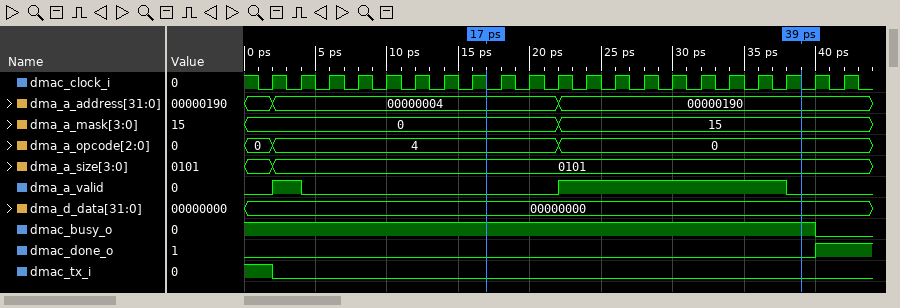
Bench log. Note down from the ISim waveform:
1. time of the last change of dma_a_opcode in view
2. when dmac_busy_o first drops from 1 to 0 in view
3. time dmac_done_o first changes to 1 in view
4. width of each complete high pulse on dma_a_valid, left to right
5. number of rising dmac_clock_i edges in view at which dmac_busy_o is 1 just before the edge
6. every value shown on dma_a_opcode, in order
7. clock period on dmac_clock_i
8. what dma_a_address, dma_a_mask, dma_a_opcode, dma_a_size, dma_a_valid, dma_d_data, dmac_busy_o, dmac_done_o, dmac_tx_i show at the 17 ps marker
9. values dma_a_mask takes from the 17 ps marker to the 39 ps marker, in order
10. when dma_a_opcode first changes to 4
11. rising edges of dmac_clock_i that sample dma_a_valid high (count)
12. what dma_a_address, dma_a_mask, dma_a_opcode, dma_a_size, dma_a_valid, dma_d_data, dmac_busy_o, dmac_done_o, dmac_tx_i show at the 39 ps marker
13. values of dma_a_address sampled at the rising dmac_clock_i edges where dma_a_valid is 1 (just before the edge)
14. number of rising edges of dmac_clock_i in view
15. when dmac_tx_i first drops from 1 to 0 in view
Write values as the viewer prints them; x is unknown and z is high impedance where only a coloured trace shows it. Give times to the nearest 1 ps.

22 ps
40 ps
40 ps
2 ps, 16 ps
20
0, 4, 0
2 ps
dma_a_address=00000004, dma_a_mask=0, dma_a_opcode=4, dma_a_size=0101, dma_a_valid=0, dma_d_data=00000000, dmac_busy_o=1, dmac_done_o=0, dmac_tx_i=0
0, 15
2 ps
9
dma_a_address=00000190, dma_a_mask=15, dma_a_opcode=0, dma_a_size=0101, dma_a_valid=0, dma_d_data=00000000, dmac_busy_o=1, dmac_done_o=0, dmac_tx_i=0
00000004, 00000190, 00000190, 00000190, 00000190, 00000190, 00000190, 00000190, 00000190
21
2 ps
